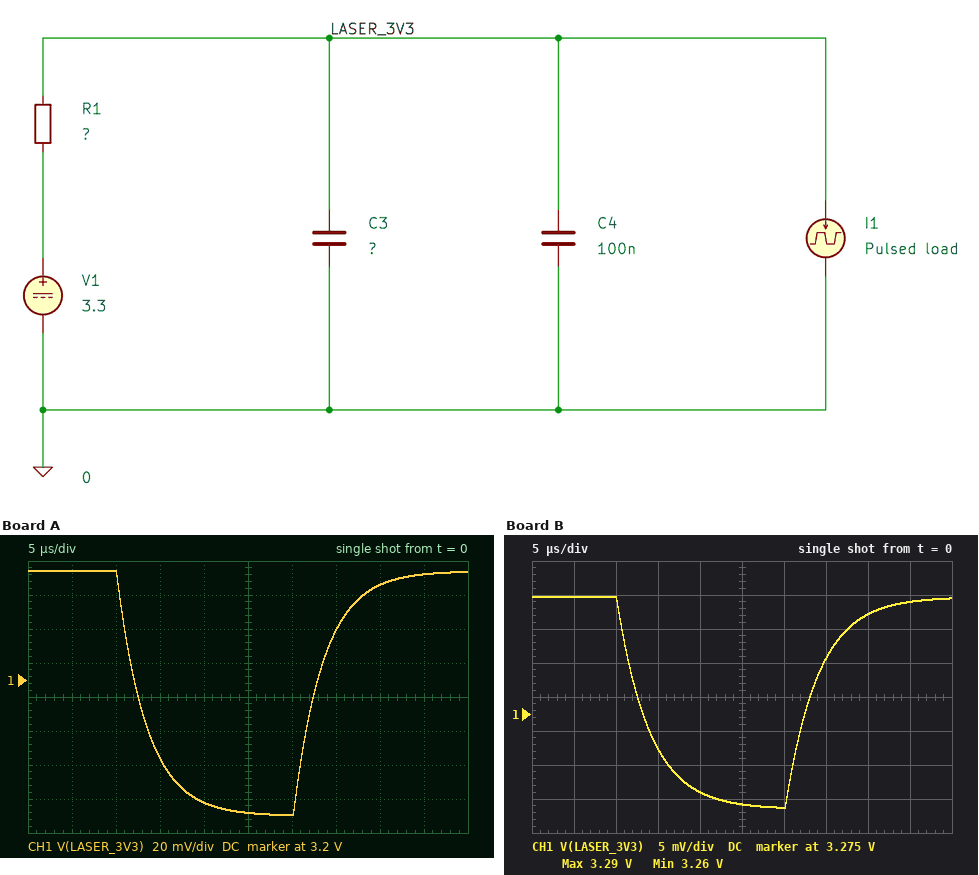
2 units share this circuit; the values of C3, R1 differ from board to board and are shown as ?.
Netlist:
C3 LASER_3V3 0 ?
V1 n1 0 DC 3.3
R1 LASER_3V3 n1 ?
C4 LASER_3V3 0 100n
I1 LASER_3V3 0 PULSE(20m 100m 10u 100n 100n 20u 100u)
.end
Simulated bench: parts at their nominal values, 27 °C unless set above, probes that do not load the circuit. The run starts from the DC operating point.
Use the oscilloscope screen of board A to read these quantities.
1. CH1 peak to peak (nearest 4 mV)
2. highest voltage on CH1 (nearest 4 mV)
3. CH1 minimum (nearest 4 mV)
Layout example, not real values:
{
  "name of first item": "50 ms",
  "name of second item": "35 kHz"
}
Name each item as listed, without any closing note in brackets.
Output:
{
  "CH1 peak to peak": "144 mV",
  "highest voltage on CH1": "3.264 V",
  "CH1 minimum": "3.120 V"
}
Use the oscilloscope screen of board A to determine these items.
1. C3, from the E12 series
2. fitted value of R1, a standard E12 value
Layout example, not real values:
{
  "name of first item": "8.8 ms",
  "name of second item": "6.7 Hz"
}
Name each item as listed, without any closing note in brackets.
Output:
{
  "C3, from the E12 series": "1.8 µF",
  "fitted value of R1, a standard E12 value": "1.8 Ω"
}
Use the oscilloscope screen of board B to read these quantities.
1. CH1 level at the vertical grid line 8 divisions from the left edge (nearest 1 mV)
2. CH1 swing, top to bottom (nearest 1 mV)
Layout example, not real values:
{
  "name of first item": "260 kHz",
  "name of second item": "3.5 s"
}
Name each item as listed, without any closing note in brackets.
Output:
{
  "CH1 level at the vertical grid line 8 divisions from the left edge": "3.290 V",
  "CH1 swing, top to bottom": "31 mV"
}
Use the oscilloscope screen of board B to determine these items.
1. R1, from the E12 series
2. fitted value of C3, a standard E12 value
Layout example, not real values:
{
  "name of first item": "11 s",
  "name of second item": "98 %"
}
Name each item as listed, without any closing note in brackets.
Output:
{
  "R1, from the E12 series": "0.39 Ω",
  "fitted value of C3, a standard E12 value": "10 µF"
}
